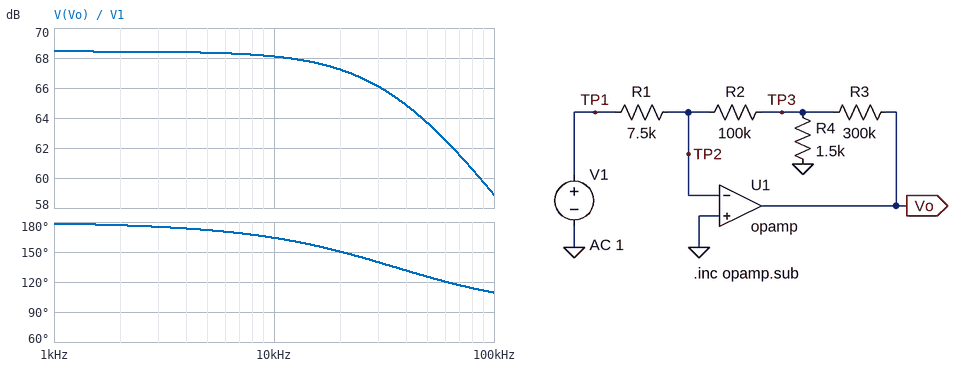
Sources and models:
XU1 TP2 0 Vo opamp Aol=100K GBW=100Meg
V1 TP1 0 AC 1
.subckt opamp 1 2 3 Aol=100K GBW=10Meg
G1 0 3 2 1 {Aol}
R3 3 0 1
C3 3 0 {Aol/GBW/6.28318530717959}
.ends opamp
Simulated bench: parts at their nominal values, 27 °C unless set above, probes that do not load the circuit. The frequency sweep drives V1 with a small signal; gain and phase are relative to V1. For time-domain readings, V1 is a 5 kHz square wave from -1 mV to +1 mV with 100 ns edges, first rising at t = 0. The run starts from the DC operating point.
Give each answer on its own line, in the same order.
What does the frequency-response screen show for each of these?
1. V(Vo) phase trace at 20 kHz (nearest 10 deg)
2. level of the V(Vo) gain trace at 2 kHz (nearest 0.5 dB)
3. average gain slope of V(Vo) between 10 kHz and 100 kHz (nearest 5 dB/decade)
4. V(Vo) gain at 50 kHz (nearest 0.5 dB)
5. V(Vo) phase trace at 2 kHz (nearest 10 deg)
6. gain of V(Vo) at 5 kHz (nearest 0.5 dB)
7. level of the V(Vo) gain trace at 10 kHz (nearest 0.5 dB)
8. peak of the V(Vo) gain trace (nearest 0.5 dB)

150 deg
68.5 dB
-10 dB/decade
63.5 dB
180 deg
68.5 dB
68.0 dB
68.5 dB
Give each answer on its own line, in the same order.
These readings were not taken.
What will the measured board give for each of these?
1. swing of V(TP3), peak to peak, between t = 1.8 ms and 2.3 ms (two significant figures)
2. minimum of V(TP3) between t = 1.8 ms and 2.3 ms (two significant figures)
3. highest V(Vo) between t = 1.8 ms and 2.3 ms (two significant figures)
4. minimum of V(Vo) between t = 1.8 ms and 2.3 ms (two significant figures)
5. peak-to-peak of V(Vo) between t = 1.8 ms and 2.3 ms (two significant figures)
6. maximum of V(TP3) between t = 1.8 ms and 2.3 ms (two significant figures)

26 mV
-13 mV
2.6 V
-2.6 V
5.3 V
13 mV
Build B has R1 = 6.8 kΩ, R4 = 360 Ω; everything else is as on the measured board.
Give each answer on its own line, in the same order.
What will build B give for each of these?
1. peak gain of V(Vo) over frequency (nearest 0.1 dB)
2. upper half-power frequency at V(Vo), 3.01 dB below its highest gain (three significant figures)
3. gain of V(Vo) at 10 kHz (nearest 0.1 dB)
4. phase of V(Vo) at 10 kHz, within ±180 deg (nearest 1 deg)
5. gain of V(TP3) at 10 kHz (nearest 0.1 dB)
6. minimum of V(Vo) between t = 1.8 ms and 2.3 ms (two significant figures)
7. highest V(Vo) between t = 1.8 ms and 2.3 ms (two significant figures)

80.7 dB
8.61 kHz
77.0 dB
131 deg
18.6 dB
-11 V
11 V
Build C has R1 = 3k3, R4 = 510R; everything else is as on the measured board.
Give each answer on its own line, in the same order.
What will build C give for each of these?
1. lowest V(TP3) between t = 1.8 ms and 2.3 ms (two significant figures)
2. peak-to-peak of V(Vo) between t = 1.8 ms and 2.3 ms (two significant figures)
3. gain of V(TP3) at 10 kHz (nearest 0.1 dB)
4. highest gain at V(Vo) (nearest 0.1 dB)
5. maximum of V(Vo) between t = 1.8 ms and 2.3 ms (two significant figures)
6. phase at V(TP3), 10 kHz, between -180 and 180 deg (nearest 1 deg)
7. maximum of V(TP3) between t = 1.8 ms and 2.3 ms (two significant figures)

-25 mV
29 V
22.8 dB
83.6 dB
15 V
123 deg
25 mV
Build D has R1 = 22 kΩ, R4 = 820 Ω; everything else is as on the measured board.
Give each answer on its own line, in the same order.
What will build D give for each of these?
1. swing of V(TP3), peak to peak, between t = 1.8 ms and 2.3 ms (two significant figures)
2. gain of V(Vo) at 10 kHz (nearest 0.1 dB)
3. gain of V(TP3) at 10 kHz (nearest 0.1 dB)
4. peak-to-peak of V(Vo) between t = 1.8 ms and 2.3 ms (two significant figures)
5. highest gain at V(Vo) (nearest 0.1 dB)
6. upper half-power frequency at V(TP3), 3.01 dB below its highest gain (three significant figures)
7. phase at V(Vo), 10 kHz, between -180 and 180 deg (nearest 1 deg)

8.9 mV
64.2 dB
12.8 dB
3.3 V
64.3 dB
49.8 kHz
169 deg
